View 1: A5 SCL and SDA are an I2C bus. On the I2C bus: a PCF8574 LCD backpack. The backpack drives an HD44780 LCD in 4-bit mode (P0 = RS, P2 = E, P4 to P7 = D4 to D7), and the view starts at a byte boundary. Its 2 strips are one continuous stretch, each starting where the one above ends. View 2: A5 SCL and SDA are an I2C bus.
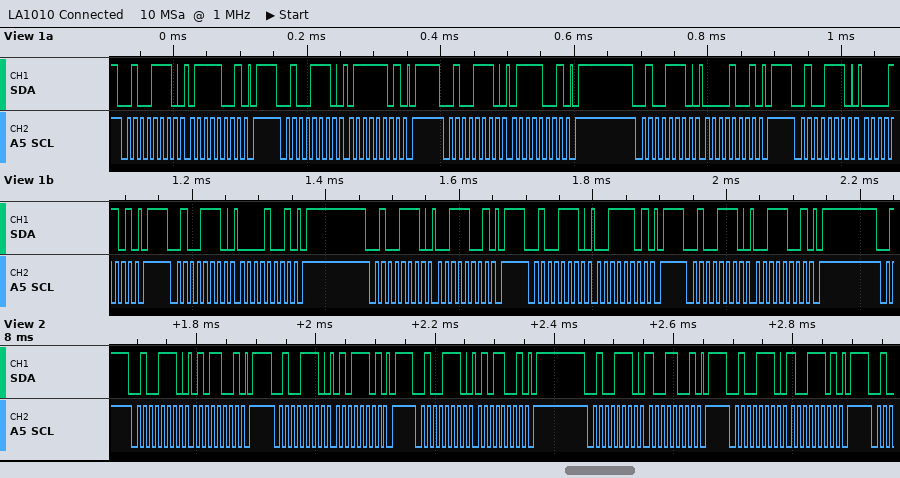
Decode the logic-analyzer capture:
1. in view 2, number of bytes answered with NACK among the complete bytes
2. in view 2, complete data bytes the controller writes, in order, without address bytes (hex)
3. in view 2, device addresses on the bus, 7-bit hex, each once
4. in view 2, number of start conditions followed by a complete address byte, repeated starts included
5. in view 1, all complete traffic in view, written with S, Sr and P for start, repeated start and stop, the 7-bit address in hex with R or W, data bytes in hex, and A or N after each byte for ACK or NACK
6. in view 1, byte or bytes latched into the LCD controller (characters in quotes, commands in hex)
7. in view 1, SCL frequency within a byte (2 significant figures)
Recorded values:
0
59 5D 59 99 9D
0x27
5
S 27W A 79 A P S 27W A 7D A P S 27W A 79 A P S 27W A 09 A P S 27W A 0D A P S 27W A 09 A P S 27W A 39 A P S 27W A 3D A P S 27W A 39 A P
'p'
100 kHz
